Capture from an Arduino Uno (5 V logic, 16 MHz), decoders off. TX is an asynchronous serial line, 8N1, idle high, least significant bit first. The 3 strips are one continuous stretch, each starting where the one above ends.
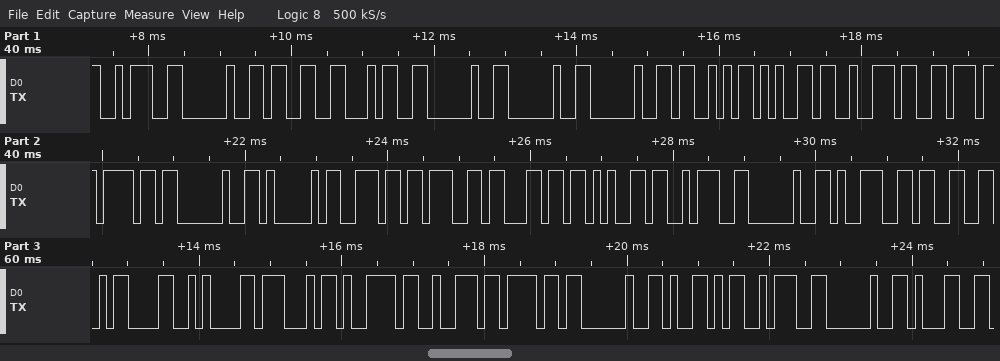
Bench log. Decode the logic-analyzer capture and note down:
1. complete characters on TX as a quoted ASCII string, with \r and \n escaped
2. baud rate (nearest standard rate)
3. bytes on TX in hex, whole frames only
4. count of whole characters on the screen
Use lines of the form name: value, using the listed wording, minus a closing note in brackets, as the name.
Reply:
complete characters on TX as a quoted ASCII string, with \r and \n escaped: ": 34   Servo Angle: 93\r\nGyro Y: 1"
baud rate: 9600 baud
bytes on TX in hex, whole frames only: 3A 20 33 34 20 20 20 53 65 72 76 6F 20 41 6E 67 6C 65 3A 20 39 33 0D 0A 47 79 72 6F 20 59 3A 20 31
count of whole characters on the screen: 33
